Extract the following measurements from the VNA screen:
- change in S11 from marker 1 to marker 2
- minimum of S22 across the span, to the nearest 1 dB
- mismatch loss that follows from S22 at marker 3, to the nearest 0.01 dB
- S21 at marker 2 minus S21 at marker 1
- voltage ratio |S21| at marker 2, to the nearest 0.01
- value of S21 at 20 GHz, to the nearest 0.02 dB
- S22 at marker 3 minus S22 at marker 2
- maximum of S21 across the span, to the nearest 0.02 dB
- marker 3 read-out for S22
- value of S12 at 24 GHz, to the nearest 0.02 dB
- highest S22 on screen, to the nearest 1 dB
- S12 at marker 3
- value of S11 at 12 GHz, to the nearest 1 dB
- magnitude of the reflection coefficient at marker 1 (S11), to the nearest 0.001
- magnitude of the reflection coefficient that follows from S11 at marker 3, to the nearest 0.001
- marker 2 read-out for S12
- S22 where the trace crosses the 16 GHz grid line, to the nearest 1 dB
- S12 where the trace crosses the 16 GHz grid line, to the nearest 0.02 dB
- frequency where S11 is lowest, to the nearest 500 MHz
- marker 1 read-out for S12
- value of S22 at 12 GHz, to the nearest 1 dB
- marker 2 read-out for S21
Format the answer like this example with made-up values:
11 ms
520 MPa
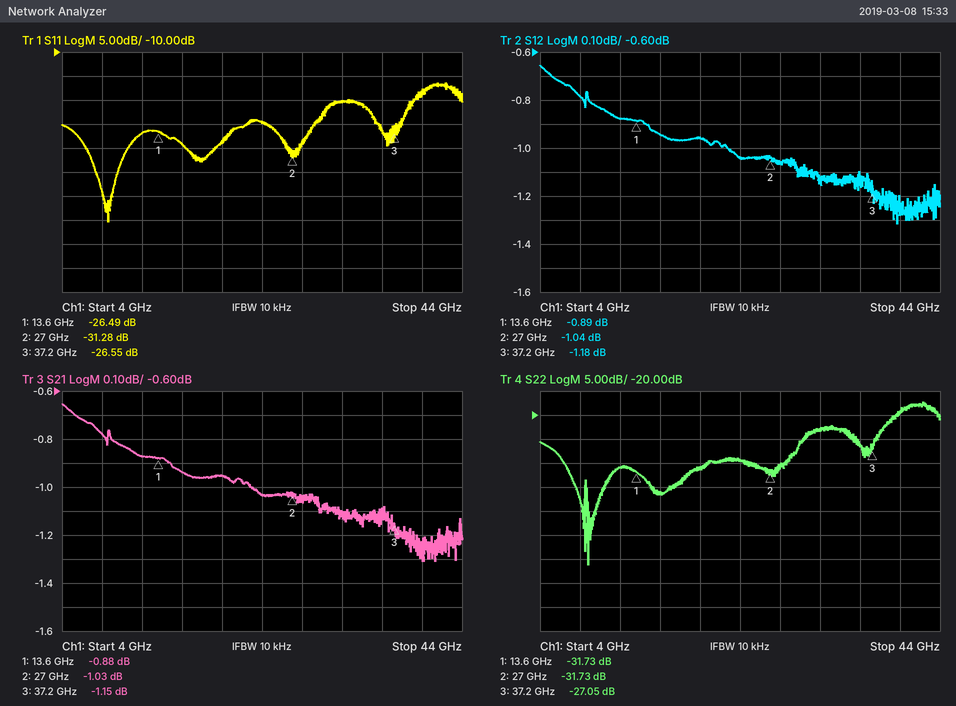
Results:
-4.79 dB
-51 dB
0.01 dB
-0.15 dB
0.89
-0.96 dB
4.68 dB
-0.66 dB
-27.05 dB
-1.04 dB
-17 dB
-1.18 dB
-27 dB
0.047
0.047
-1.04 dB
-36 dB
-0.94 dB
8.5 GHz
-0.89 dB
-31 dB
-1.03 dB
